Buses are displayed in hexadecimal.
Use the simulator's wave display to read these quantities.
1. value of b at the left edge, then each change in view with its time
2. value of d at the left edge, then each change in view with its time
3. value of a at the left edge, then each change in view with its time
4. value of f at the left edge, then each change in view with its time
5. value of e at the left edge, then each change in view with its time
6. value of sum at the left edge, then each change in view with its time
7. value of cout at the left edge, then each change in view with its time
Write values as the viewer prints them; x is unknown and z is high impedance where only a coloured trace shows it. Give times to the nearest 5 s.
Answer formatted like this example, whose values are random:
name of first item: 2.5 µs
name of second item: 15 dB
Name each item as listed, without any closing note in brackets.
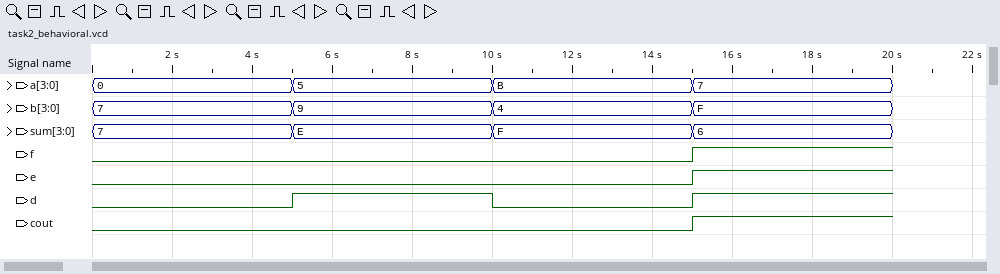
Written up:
value of b at the left edge, then each change in view with its time: 7, 9 at 5 s, 4 at 10 s, F at 15 s
value of d at the left edge, then each change in view with its time: 0, 1 at 5 s, 0 at 10 s, 1 at 15 s
value of a at the left edge, then each change in view with its time: 0, 5 at 5 s, B at 10 s, 7 at 15 s
value of f at the left edge, then each change in view with its time: 0, 1 at 15 s
value of e at the left edge, then each change in view with its time: 0, 1 at 15 s
value of sum at the left edge, then each change in view with its time: 7, E at 5 s, F at 10 s, 6 at 15 s
value of cout at the left edge, then each change in view with its time: 0, 1 at 15 s
